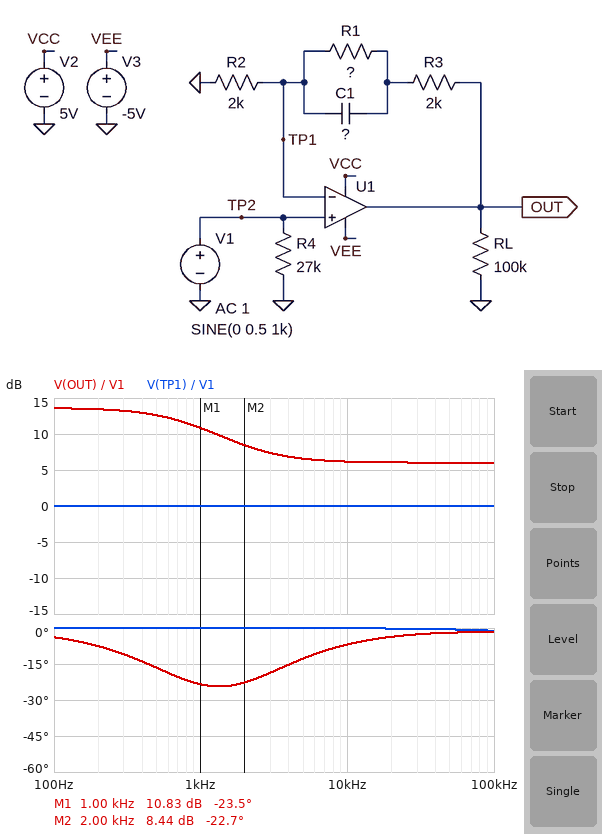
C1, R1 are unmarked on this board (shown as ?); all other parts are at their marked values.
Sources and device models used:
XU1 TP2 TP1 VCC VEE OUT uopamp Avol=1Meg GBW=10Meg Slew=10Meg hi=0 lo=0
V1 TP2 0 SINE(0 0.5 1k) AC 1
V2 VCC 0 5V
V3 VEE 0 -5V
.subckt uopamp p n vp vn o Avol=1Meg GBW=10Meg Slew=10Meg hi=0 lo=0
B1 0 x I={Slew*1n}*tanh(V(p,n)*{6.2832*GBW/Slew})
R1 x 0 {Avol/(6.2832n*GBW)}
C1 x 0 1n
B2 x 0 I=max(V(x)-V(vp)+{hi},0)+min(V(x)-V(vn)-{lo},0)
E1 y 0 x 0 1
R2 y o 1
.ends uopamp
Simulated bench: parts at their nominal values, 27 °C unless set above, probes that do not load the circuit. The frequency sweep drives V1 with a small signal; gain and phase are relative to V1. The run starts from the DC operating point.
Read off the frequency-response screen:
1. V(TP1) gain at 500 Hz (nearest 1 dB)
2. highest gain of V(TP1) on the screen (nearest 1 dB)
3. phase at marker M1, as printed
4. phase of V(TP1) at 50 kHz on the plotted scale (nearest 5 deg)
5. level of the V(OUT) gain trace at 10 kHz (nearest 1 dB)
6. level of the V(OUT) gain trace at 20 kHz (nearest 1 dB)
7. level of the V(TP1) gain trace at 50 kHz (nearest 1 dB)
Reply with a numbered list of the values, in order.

1. 0 dB
2. 0 dB
3. -23.5 deg
4. 0 deg
5. 6 dB
6. 6 dB
7. 0 dB
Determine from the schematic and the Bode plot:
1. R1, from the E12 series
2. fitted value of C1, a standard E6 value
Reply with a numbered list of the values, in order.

1. 5.6 kΩ
2. 33 nF
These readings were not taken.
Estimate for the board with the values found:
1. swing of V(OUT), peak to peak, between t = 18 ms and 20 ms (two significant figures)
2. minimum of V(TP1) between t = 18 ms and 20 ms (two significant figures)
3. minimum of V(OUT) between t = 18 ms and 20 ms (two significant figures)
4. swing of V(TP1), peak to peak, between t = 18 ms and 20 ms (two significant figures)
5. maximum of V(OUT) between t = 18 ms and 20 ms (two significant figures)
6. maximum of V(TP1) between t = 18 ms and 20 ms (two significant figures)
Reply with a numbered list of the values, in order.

1. 3.5 V
2. -500 mV
3. -1.7 V
4. 1.0 V
5. 1.7 V
6. 500 mV
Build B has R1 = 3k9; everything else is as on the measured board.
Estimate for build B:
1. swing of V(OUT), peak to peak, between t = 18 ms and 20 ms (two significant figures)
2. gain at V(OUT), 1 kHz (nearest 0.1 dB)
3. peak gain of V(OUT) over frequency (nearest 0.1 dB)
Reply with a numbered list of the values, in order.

1. 3.3 V
2. 10.4 dB
3. 11.9 dB
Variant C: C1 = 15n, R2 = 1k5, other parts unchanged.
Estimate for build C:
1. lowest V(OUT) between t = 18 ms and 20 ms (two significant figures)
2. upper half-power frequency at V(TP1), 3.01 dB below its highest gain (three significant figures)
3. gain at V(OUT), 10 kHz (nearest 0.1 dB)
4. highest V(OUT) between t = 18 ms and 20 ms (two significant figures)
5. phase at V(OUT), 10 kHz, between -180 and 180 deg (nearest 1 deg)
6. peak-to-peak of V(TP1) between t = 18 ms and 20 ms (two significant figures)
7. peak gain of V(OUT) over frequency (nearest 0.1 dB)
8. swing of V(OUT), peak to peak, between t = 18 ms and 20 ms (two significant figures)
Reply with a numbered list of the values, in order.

1. -2.7 V
2. 4.28 MHz
3. 8.1 dB
4. 2.7 V
5. -16 deg
6. 1.0 V
7. 15.7 dB
8. 5.5 V
